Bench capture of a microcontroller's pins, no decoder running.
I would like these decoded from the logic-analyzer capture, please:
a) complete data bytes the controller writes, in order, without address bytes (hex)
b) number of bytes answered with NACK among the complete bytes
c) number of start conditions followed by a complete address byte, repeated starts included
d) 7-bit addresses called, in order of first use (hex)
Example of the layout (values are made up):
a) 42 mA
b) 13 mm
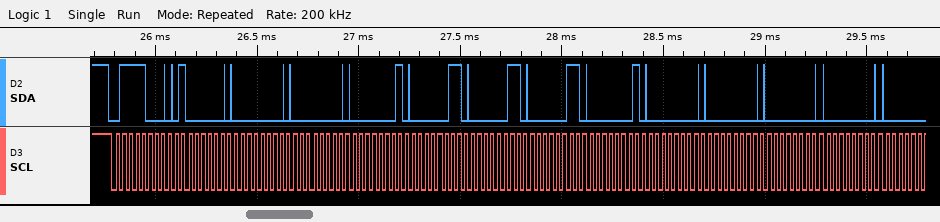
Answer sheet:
a) 40 00 00 01 03 03 03 01 00 00 00 00
b) 0
c) 1
d) 0x3C
